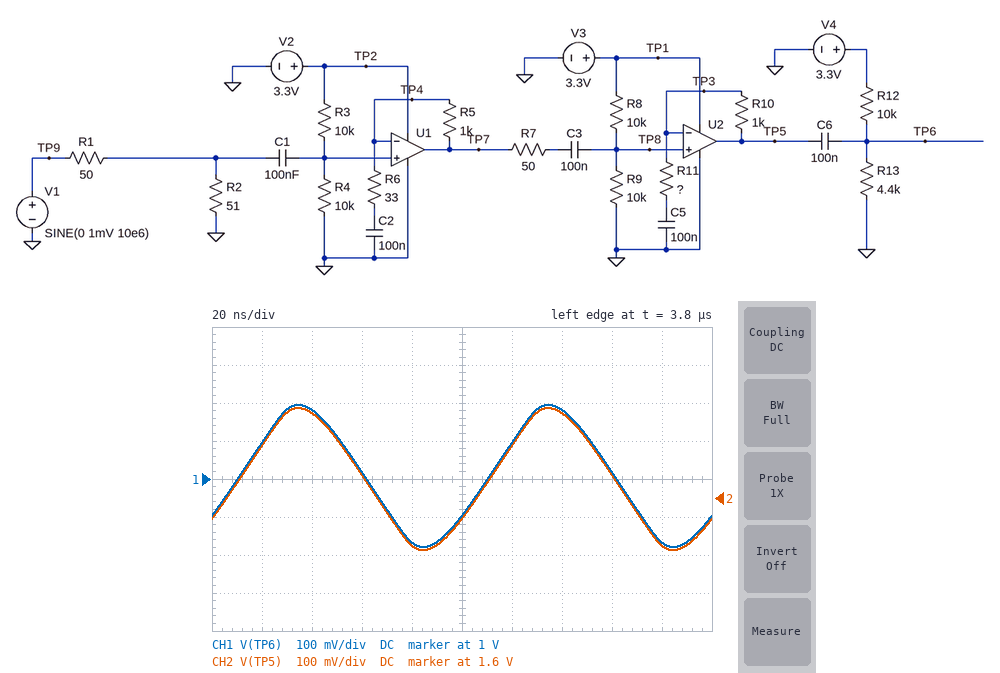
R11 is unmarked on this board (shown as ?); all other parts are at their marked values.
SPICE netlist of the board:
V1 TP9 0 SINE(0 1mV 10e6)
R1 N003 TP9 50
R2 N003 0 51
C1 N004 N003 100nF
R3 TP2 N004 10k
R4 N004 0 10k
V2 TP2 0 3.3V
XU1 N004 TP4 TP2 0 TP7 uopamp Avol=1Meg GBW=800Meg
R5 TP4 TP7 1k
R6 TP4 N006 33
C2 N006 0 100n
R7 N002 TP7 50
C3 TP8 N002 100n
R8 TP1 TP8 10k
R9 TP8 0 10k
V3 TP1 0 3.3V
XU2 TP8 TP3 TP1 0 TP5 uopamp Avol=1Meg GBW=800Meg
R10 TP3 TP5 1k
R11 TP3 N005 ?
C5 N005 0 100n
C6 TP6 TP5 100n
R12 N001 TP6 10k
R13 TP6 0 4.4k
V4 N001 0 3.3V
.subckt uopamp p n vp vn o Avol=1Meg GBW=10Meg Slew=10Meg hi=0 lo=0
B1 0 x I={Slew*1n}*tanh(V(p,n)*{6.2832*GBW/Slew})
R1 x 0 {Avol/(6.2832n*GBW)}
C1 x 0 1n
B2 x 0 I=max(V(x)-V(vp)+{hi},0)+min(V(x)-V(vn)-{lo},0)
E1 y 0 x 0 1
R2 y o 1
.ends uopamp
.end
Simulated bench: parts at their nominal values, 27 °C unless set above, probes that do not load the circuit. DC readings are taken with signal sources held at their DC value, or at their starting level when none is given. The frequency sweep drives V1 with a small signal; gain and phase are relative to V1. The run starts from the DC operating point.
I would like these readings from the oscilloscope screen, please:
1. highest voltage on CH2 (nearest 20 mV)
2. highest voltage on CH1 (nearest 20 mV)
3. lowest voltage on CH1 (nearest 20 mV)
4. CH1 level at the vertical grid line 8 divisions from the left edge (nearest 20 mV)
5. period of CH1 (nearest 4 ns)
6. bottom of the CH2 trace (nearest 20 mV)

1.84 V
1.20 V
820 mV
1.02 V
100 ns
1.46 V
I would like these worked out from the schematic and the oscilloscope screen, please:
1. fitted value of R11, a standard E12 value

82 Ω
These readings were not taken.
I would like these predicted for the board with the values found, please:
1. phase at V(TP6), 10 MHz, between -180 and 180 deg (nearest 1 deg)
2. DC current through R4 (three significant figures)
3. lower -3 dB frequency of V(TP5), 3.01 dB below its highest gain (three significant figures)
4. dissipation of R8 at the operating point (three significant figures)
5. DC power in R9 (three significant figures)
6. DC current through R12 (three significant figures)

-30 deg
165 µA
54.5 kHz
272 µW
272 µW
229 µA
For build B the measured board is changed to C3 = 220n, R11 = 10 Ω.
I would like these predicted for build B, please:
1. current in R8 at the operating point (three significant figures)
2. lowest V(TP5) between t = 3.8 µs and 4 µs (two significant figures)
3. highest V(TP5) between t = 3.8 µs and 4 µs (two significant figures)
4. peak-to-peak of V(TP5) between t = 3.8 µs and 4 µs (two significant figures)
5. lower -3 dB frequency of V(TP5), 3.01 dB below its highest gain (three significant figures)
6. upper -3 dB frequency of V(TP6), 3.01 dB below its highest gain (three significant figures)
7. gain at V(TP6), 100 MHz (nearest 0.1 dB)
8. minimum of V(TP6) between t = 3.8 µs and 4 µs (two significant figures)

165 µA
1.4 V
1.9 V
470 mV
168 kHz
7.46 MHz
29.7 dB
770 mV
